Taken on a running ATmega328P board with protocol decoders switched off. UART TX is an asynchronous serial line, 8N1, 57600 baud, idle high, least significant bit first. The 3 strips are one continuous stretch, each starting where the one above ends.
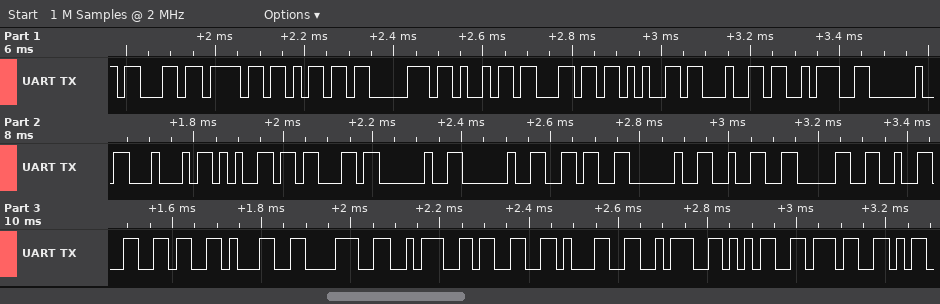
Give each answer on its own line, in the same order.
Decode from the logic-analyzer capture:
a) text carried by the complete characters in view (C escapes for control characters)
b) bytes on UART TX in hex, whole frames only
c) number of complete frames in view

"compiled: Dec  6 202618:31:57"
0x63 0x6F 0x6D 0x70 0x69 0x6C 0x65 0x64 0x3A 0x20 0x44 0x65 0x63 0x20 0x20 0x36 0x20 0x32 0x30 0x32 0x36 0x31 0x38 0x3A 0x33 0x31 0x3A 0x35 0x37
29
